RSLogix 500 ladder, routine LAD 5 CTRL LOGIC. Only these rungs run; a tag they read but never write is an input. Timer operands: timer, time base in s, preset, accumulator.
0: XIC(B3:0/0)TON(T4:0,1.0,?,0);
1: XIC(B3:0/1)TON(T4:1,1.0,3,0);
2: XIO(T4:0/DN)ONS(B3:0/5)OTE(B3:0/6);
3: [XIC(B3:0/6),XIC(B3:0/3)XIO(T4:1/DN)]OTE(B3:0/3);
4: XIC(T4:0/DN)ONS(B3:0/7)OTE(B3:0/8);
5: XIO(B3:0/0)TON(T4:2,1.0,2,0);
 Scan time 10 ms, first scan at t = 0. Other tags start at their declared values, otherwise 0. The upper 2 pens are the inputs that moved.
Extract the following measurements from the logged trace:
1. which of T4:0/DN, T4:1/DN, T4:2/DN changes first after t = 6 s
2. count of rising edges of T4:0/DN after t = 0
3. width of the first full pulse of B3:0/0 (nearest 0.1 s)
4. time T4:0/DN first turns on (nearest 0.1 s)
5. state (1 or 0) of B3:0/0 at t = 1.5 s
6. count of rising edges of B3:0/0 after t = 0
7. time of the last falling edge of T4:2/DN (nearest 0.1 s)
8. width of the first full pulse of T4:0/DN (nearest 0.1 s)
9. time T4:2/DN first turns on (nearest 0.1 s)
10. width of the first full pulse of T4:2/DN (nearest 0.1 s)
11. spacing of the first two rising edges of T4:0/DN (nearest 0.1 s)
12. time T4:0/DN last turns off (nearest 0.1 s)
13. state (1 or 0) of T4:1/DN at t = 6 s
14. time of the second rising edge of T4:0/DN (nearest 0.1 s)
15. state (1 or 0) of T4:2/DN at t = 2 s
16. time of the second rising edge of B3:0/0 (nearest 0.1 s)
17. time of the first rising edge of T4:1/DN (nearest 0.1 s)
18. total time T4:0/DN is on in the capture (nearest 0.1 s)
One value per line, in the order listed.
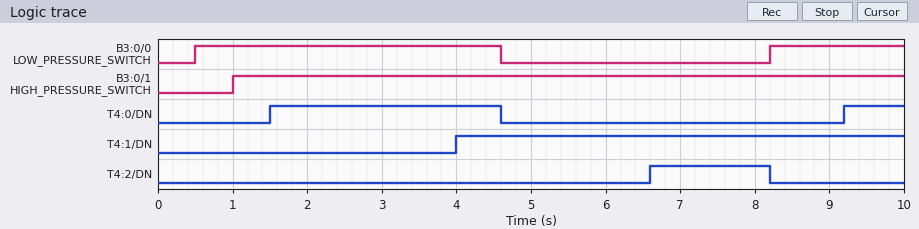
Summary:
T4:2/DN
2
4.1 s
1.5 s
1
2
8.2 s
3.1 s
6.6 s
1.6 s
7.7 s
4.6 s
1
9.2 s
0
8.2 s
4.0 s
3.9 s
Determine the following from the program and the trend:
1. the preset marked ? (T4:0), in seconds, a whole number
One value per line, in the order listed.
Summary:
1 s
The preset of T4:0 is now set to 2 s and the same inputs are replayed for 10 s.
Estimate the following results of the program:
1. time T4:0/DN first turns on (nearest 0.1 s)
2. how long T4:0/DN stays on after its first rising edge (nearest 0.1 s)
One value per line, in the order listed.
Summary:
2.5 s
2.1 s
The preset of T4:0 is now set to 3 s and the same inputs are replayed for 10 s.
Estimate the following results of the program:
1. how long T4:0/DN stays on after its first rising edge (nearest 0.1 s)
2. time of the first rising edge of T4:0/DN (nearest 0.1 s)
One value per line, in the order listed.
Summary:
1.1 s
3.5 s
